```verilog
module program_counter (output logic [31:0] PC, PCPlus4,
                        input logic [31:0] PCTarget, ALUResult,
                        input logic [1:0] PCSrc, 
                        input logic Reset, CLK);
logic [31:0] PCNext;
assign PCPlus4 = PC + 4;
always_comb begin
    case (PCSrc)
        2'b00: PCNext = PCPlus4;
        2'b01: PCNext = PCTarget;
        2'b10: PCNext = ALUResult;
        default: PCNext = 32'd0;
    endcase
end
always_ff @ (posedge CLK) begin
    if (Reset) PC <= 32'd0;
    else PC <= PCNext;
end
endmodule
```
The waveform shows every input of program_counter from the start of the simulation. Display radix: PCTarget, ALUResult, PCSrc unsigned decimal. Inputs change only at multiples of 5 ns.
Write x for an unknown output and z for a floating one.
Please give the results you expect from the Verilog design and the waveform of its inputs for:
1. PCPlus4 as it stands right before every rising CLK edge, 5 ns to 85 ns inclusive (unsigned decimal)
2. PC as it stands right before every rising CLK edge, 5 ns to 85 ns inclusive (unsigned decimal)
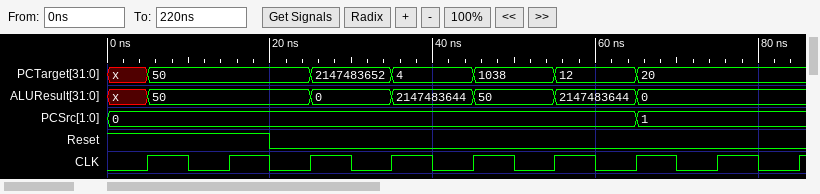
x, 4, 4, 8, 12, 16, 20, 24, 24
x, 0, 0, 4, 8, 12, 16, 20, 20
